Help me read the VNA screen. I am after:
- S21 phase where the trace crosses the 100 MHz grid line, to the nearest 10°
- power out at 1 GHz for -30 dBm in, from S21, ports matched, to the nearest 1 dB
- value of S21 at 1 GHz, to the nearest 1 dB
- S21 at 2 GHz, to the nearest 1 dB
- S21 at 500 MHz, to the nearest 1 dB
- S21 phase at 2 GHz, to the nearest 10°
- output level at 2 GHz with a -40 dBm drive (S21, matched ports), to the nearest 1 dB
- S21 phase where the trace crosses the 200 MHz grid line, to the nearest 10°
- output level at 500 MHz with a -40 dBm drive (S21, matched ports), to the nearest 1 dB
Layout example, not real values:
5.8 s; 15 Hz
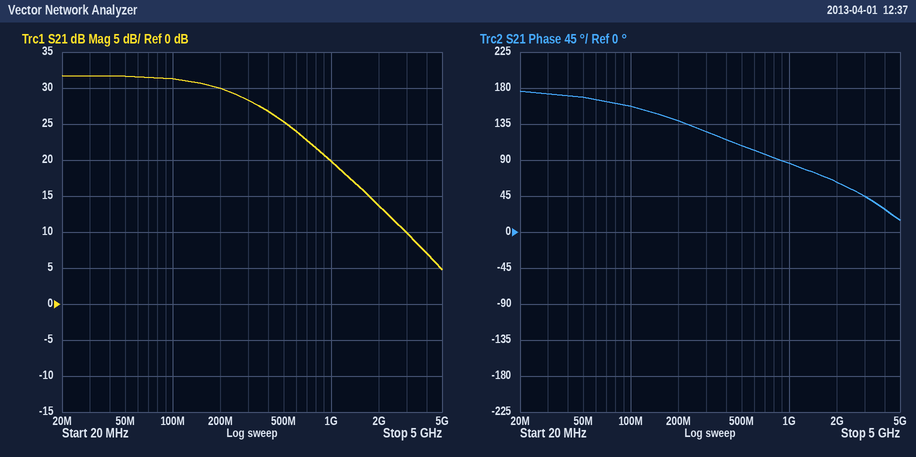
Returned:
160°; -10 dBm; 20 dB; 14 dB; 25 dB; 60°; -26 dBm; 140°; -15 dBm
